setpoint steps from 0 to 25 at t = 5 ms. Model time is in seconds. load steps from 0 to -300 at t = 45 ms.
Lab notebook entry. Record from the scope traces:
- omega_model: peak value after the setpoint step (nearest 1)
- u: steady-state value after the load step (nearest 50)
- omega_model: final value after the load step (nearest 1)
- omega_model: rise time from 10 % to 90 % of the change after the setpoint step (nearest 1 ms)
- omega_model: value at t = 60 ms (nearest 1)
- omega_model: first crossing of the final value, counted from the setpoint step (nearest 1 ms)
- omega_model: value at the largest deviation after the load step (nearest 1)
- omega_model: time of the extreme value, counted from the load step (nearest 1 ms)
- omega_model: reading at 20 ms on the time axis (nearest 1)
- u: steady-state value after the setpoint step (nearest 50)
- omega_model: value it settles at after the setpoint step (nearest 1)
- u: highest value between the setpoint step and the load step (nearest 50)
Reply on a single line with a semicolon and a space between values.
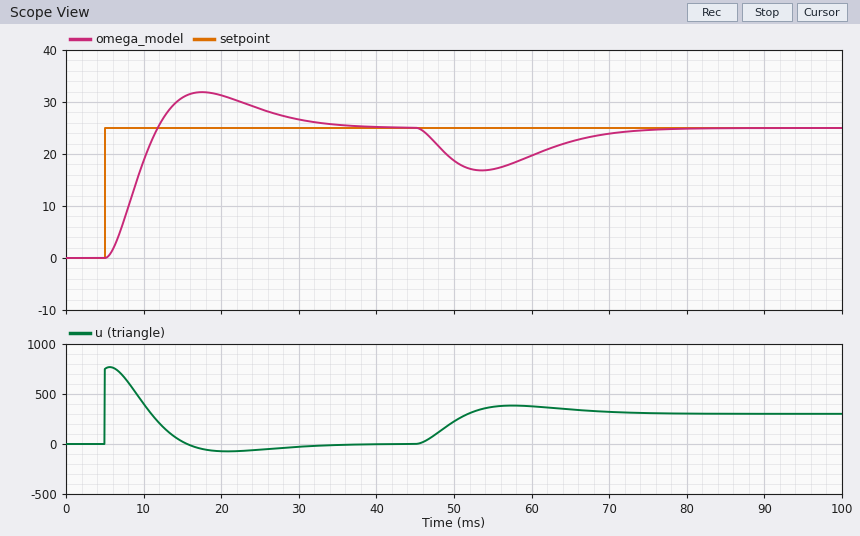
32; 300; 25; 5 ms; 20; 7 ms; 17; 9 ms; 31; 0; 25; 750
